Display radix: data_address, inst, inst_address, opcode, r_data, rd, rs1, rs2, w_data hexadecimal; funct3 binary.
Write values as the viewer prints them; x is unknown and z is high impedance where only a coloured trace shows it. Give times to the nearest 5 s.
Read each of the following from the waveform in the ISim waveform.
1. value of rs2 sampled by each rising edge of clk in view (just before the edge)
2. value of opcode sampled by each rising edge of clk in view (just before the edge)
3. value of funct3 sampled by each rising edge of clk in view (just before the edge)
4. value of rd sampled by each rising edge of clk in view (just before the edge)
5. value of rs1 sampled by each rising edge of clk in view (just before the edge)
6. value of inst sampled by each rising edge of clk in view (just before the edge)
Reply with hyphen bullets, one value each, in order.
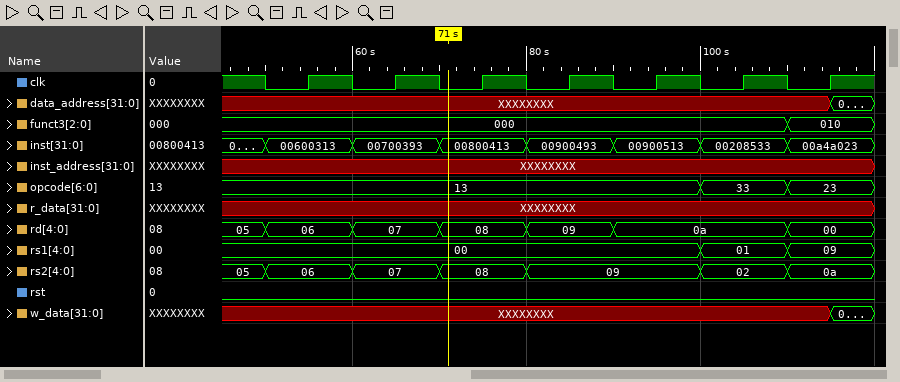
- 06, 07, 08, 09, 09, 02, 0a
- 13, 13, 13, 13, 13, 33, 23
- 000, 000, 000, 000, 000, 000, 010
- 06, 07, 08, 09, 0a, 0a, 00
- 00, 00, 00, 00, 00, 01, 09
- 00600313, 00700393, 00800413, 00900493, 00900513, 00208533, 00a4a023
